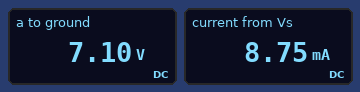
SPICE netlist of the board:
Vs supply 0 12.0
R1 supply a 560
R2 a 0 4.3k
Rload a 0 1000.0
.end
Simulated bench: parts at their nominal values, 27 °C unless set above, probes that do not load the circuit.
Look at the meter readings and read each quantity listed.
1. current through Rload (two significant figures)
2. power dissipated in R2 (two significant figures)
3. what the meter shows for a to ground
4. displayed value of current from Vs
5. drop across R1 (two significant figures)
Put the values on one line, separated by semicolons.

7.1 mA; 12 mW; 7.10 V; 8.75 mA; 4.9 V
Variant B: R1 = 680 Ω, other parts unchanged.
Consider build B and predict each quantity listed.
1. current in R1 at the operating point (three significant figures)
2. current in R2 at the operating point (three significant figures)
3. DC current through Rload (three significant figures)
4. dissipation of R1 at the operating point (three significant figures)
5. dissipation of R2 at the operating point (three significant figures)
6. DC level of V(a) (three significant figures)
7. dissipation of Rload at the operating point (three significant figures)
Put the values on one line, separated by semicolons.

8.05 mA; 1.52 mA; 6.53 mA; 44.0 mW; 9.91 mW; 6.53 V; 42.6 mW
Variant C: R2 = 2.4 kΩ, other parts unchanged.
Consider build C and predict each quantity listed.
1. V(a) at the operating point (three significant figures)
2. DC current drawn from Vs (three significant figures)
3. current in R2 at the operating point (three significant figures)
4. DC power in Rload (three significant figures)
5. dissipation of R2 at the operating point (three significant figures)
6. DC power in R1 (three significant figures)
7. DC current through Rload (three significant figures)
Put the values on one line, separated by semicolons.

6.69 V; 9.48 mA; 2.79 mA; 44.8 mW; 18.7 mW; 50.3 mW; 6.69 mA
